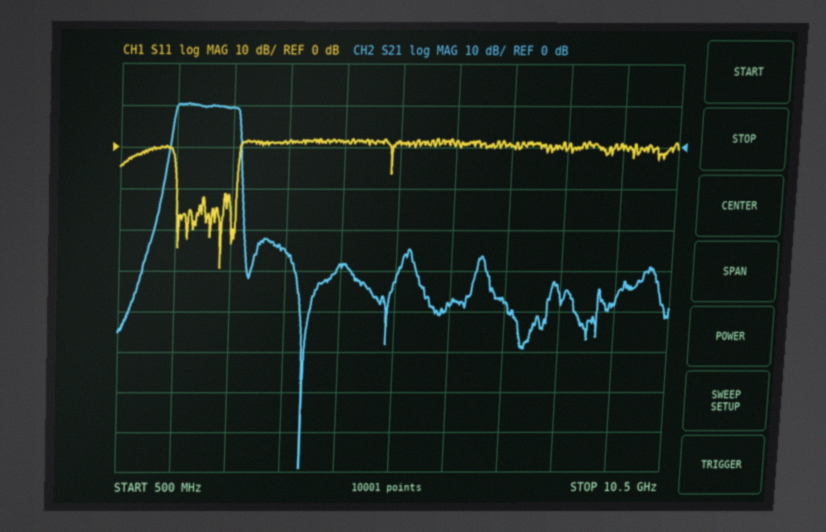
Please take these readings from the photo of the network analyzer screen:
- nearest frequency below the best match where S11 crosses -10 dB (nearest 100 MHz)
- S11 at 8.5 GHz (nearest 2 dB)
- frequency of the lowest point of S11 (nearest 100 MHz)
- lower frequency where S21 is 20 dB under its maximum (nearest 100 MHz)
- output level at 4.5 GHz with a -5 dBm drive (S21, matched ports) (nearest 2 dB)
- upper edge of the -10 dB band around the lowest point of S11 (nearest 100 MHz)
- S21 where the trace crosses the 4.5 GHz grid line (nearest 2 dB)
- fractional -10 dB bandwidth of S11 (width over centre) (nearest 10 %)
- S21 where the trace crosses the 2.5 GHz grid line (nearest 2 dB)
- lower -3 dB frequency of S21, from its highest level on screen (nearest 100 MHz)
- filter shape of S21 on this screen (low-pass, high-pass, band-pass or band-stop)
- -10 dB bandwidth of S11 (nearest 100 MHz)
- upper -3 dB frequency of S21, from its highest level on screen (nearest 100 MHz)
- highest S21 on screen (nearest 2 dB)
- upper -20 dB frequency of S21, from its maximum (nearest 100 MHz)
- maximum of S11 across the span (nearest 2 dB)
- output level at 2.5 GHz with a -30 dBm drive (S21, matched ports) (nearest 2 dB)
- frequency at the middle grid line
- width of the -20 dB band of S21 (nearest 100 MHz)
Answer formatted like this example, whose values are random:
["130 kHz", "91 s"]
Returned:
["1.5 GHz", "0 dB", "2.3 GHz", "1.3 GHz", "-34 dBm", "2.6 GHz", "-28 dB", "50 %", "10 dB", "1.5 GHz", "band-pass", "1.1 GHz", "2.6 GHz", "10 dB", "2.7 GHz", "2 dB", "-20 dBm", "5.5 GHz", "1.4 GHz"]
